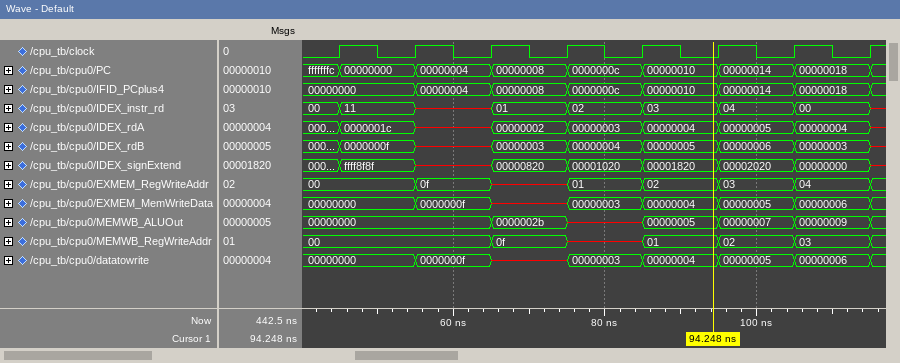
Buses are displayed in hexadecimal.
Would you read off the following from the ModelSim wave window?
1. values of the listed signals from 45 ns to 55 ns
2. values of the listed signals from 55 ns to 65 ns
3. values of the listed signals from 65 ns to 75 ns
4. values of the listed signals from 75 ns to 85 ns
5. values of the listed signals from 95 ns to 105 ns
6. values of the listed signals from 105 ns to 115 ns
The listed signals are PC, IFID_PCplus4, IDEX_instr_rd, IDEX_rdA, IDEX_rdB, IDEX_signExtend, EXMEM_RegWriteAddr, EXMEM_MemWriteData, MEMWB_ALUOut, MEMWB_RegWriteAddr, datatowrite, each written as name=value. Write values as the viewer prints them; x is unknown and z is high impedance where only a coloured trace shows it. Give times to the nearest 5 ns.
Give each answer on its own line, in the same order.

PC=00000000, IFID_PCplus4=00000000, IDEX_instr_rd=11, IDEX_rdA=0000001c, IDEX_rdB=0000000f, IDEX_signExtend=ffff8f8f, EXMEM_RegWriteAddr=00, EXMEM_MemWriteData=00000000, MEMWB_ALUOut=00000000, MEMWB_RegWriteAddr=00, datatowrite=00000000
PC=00000004, IFID_PCplus4=00000004, IDEX_instr_rd=x, IDEX_rdA=x, IDEX_rdB=x, IDEX_signExtend=x, EXMEM_RegWriteAddr=0f, EXMEM_MemWriteData=0000000f, MEMWB_ALUOut=00000000, MEMWB_RegWriteAddr=00, datatowrite=0000000f
PC=00000008, IFID_PCplus4=00000008, IDEX_instr_rd=01, IDEX_rdA=00000002, IDEX_rdB=00000003, IDEX_signExtend=00000820, EXMEM_RegWriteAddr=x, EXMEM_MemWriteData=x, MEMWB_ALUOut=0000002b, MEMWB_RegWriteAddr=0f, datatowrite=x
PC=0000000c, IFID_PCplus4=0000000c, IDEX_instr_rd=02, IDEX_rdA=00000003, IDEX_rdB=00000004, IDEX_signExtend=00001020, EXMEM_RegWriteAddr=01, EXMEM_MemWriteData=00000003, MEMWB_ALUOut=x, MEMWB_RegWriteAddr=x, datatowrite=00000003
PC=00000014, IFID_PCplus4=00000014, IDEX_instr_rd=04, IDEX_rdA=00000005, IDEX_rdB=00000006, IDEX_signExtend=00002020, EXMEM_RegWriteAddr=03, EXMEM_MemWriteData=00000005, MEMWB_ALUOut=00000007, MEMWB_RegWriteAddr=02, datatowrite=00000005
PC=00000018, IFID_PCplus4=00000018, IDEX_instr_rd=00, IDEX_rdA=00000004, IDEX_rdB=00000003, IDEX_signExtend=00000000, EXMEM_RegWriteAddr=04, EXMEM_MemWriteData=00000006, MEMWB_ALUOut=00000009, MEMWB_RegWriteAddr=03, datatowrite=00000006
